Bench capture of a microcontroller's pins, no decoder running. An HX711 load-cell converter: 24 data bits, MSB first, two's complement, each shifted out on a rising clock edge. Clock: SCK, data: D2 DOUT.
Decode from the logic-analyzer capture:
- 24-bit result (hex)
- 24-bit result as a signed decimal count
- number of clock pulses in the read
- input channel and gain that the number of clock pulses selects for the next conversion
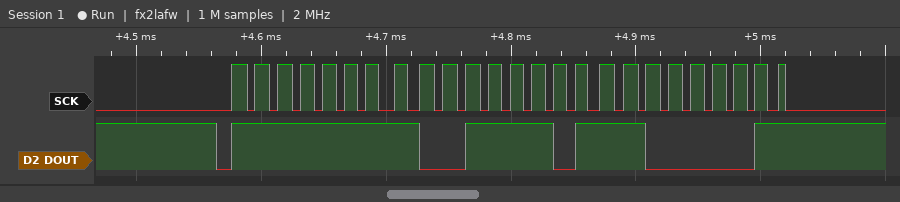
0xFF3DC1
-49727
25
channel A, gain 128
